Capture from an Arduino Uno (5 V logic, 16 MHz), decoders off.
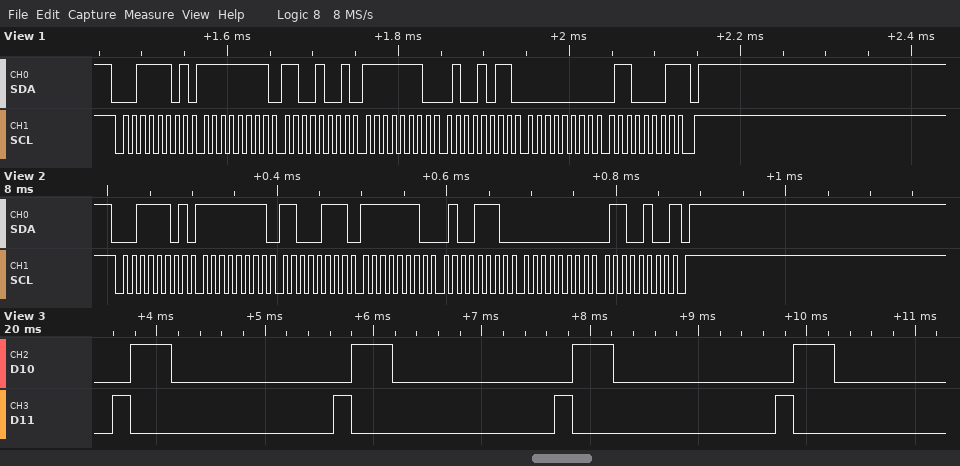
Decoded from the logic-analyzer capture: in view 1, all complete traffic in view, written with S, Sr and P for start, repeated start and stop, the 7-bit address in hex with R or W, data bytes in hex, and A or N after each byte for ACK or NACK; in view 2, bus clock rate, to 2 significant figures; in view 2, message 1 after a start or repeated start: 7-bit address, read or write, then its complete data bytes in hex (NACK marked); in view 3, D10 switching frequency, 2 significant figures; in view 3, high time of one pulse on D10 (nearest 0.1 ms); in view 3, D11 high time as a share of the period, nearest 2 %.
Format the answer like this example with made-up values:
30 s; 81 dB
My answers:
S 1ER A FF A C9 A FE A 4B A 00 A 61 N P; 100 kHz; 0x1E read: FF C7 FE 4E 00 64 NACK; 490 Hz; 0.4 ms; 8 %
